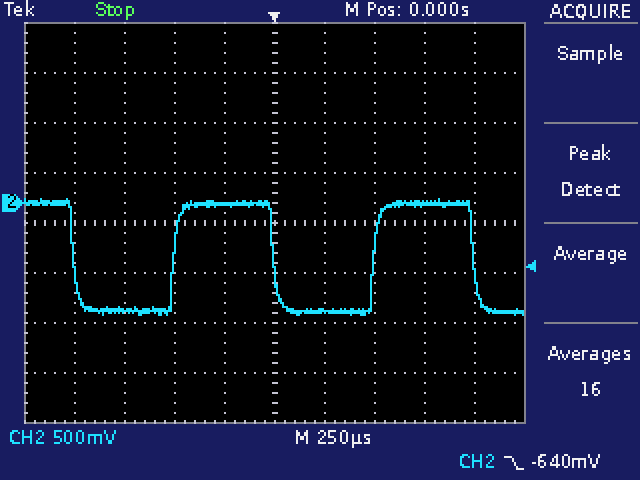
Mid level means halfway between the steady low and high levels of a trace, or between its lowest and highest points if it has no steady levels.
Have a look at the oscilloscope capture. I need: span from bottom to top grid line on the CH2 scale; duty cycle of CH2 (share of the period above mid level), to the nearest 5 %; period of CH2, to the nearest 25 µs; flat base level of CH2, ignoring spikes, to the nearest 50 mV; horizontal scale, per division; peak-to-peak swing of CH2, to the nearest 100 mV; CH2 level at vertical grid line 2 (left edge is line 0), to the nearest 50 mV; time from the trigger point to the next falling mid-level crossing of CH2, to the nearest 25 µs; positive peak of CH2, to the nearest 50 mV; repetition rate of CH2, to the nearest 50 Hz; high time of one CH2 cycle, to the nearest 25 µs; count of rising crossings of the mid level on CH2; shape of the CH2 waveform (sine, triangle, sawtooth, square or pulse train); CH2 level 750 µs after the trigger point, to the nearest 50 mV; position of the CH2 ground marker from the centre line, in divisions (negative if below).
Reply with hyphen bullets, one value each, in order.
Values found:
- 4 V
- 50 %
- 1.000 ms
- -1.10 V
- 250 µs
- 1.20 V
- -1.10 V
- 1.000 ms
- 50 mV
- 1.00 kHz
- 500 µs
- 2
- square
- 0 mV
- +0.4 div
